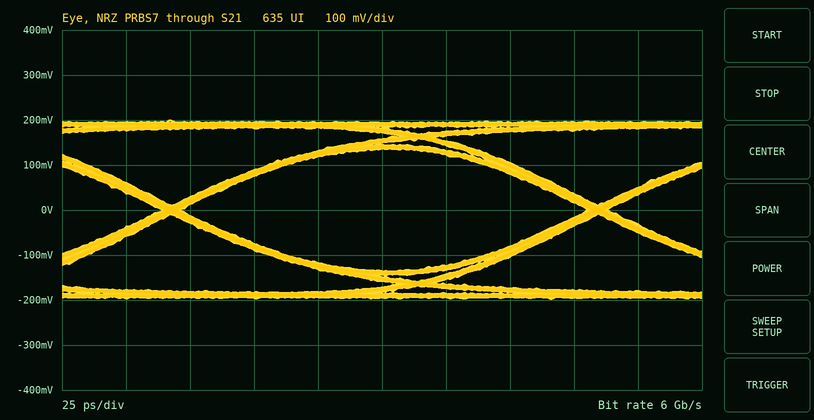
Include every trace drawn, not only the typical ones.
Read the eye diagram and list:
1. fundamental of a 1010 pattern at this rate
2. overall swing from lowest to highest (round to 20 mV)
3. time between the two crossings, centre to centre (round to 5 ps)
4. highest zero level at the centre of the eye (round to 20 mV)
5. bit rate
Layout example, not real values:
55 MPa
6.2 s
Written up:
3 GHz
400 mV
165 ps
-140 mV
6 Gb/s
